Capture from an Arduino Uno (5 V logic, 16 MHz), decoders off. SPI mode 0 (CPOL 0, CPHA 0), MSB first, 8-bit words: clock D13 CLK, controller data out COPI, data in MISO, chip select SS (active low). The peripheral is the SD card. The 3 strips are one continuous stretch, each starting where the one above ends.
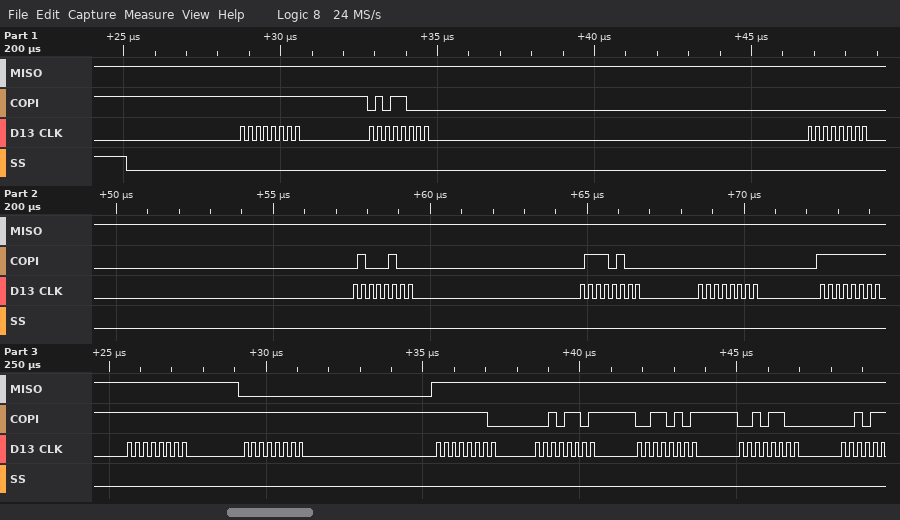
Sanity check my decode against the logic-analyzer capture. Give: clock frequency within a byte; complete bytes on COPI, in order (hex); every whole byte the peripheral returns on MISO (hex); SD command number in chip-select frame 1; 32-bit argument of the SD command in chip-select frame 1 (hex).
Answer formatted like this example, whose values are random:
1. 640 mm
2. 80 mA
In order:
1. 4 MHz
2. FF 58 00 44 74 00 FF FF FF FE 2D 35 2C
3. FF FF FF FF FF FF FF FF 00 FF FF FF FF
4. CMD24
5. 0x00447400
